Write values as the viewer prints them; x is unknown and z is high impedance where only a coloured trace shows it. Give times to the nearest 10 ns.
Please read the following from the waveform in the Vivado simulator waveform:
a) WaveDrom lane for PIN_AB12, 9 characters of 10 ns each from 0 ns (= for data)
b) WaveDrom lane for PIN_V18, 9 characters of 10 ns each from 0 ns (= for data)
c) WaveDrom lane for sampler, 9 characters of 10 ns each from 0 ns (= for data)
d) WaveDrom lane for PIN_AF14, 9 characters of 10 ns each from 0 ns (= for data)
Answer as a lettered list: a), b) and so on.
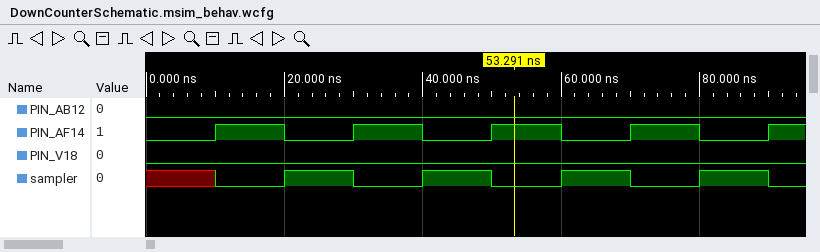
a) {name: 'PIN_AB12', wave: '0........'}
b) {name: 'PIN_V18', wave: '0........'}
c) {name: 'sampler', wave: 'x01010101'}
d) {name: 'PIN_AF14', wave: '010101010'}
